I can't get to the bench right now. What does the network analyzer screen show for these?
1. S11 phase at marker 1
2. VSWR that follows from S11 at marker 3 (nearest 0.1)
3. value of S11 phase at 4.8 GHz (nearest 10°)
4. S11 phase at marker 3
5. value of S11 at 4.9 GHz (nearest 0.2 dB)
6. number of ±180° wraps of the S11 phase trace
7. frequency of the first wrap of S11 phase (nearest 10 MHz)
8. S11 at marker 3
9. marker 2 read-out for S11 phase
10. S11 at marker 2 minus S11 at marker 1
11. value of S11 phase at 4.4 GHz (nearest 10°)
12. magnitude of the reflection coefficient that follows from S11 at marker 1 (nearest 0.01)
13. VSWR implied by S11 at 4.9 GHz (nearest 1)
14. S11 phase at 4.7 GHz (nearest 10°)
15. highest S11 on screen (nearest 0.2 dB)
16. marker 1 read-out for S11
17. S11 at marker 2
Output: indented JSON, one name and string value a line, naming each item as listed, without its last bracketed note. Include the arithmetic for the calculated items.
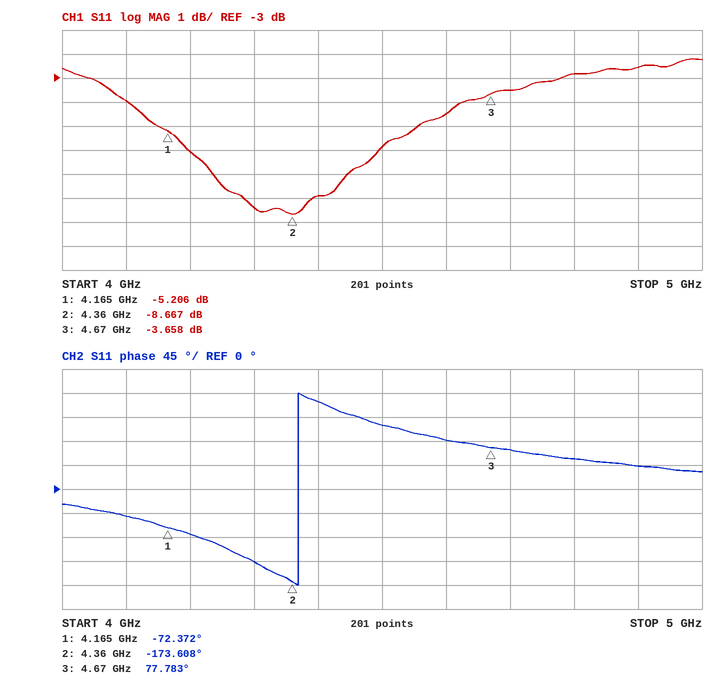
{
  "S11 phase at marker 1": "-72.372°",
  "VSWR that follows from S11 at marker 3": "(1 + 0.6563)/(1 − 0.6563) ≈ 4.8",
  "value of S11 phase at 4.8 GHz": "60°",
  "S11 phase at marker 3": "77.783°",
  "value of S11 at 4.9 GHz": "-2.6 dB",
  "number of ±180° wraps of the S11 phase trace": "1",
  "frequency of the first wrap of S11 phase": "4.37 GHz",
  "S11 at marker 3": "-3.658 dB",
  "marker 2 read-out for S11 phase": "-173.608°",
  "S11 at marker 2 minus S11 at marker 1": "-8.667 − (-5.206) = -3.461 dB",
  "value of S11 phase at 4.4 GHz": "160°",
  "magnitude of the reflection coefficient that follows from S11 at marker 1": "10^(-5.206/20) ≈ 0.55",
  "VSWR implied by S11 at 4.9 GHz": "|Γ| = 10^(-2.6/20) = 0.7413; VSWR = (1 + 0.7413)/(1 − 0.7413) ≈ 7",
  "S11 phase at 4.7 GHz": "70°",
  "highest S11 on screen": "-2.2 dB",
  "marker 1 read-out for S11": "-5.206 dB",
  "S11 at marker 2": "-8.667 dB"
}
